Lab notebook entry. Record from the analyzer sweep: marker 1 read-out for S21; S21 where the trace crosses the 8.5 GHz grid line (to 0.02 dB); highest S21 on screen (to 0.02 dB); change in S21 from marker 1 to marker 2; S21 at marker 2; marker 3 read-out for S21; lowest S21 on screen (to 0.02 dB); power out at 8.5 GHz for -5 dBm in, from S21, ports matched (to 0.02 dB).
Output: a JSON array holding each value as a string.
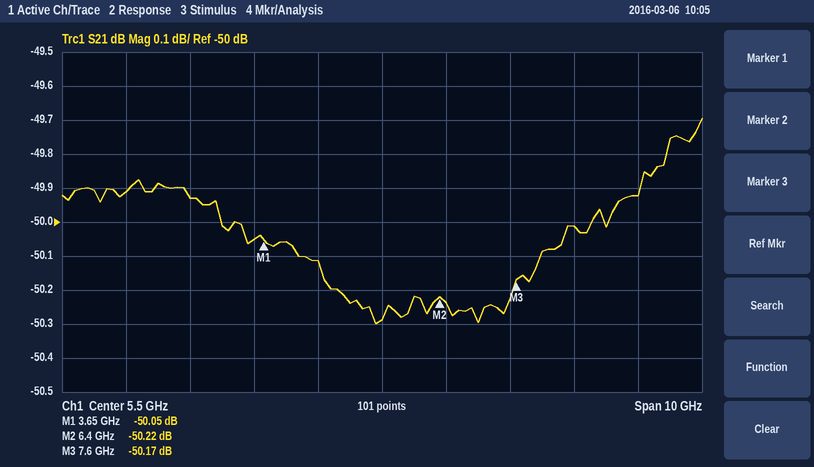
["-50.05 dB", "-50.02 dB", "-49.70 dB", "-0.17 dB", "-50.22 dB", "-50.17 dB", "-50.30 dB", "-55.02 dBm"]
